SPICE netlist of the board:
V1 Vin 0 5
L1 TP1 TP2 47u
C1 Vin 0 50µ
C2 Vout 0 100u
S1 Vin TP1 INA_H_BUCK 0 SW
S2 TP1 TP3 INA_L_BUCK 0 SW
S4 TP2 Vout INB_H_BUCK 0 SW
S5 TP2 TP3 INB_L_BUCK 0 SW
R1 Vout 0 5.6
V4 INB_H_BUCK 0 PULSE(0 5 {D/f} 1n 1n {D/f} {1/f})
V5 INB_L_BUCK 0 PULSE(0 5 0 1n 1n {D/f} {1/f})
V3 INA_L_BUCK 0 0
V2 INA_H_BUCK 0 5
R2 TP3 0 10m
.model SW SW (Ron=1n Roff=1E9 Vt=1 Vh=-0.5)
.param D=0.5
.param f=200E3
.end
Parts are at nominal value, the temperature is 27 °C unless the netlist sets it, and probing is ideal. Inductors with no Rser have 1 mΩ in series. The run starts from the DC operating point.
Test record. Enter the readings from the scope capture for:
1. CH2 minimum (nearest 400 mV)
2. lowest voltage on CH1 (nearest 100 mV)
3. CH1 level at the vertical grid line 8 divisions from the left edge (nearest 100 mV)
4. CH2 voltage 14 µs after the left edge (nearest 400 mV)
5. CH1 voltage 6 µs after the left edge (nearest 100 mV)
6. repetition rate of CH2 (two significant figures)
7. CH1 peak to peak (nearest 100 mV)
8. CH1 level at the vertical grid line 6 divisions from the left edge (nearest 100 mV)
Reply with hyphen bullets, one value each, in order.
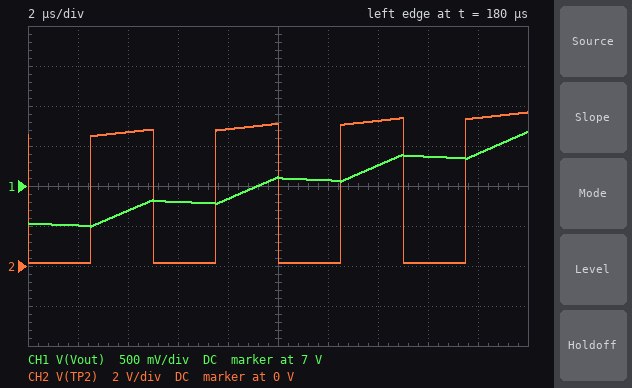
- 0 V
- 6.5 V
- 7.4 V
- 7.2 V
- 6.8 V
- 200 kHz
- 1.2 V
- 7.1 V
